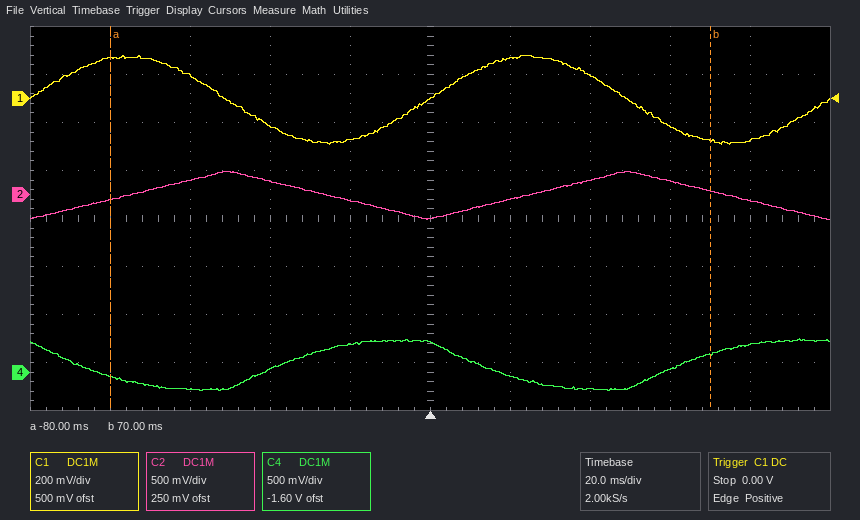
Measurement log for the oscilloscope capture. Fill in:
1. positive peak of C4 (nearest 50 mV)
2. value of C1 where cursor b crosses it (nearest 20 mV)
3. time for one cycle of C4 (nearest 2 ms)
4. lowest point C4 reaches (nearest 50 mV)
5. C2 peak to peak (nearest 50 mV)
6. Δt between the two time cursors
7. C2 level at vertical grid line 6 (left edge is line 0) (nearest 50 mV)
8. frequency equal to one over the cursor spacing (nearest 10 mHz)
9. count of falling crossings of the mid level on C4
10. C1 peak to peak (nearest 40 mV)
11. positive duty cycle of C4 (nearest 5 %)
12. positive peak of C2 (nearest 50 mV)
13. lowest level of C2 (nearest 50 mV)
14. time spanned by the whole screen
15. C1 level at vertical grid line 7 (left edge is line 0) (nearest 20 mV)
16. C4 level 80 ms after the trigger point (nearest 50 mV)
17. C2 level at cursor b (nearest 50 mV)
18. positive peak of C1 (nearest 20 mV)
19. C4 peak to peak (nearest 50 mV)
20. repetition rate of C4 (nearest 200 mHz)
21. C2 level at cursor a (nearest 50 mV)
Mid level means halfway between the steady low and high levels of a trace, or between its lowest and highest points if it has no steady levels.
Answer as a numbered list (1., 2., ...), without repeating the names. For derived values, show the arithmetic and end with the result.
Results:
1. 350 mV
2. -180 mV
3. 100 ms
4. -200 mV
5. 250 mV − (-250 mV) = 500 mV
6. 70 ms − (-80 ms) = 150 ms
7. -50 mV
8. 1 / 150 ms ≈ 6.67 Hz
9. 2
10. 360 mV
11. 50 %
12. 250 mV
13. -250 mV
14. 200 ms
15. 100 mV
16. 300 mV
17. 50 mV
18. 180 mV
19. 350 mV − (-200 mV) = 550 mV
20. 1 / 100 ms ≈ 10.0 Hz
21. -50 mV
